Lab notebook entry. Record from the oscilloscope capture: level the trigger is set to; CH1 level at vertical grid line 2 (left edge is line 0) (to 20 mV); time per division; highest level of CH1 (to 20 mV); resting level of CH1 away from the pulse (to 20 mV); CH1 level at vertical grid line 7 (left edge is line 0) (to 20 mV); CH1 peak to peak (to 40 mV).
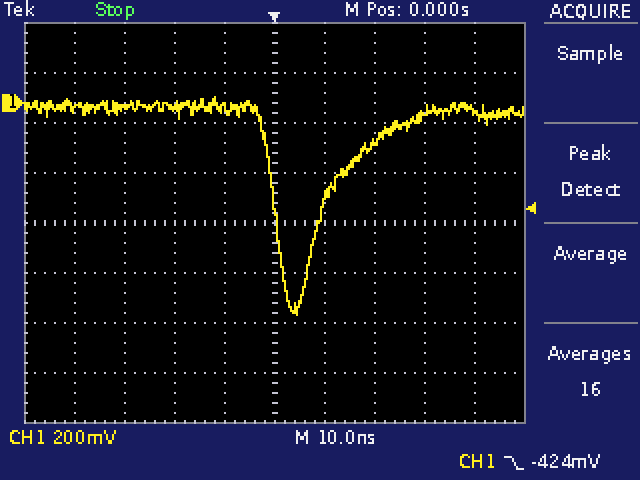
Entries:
-424 mV
-20 mV
10 ns
20 mV
-20 mV
-160 mV
880 mV
